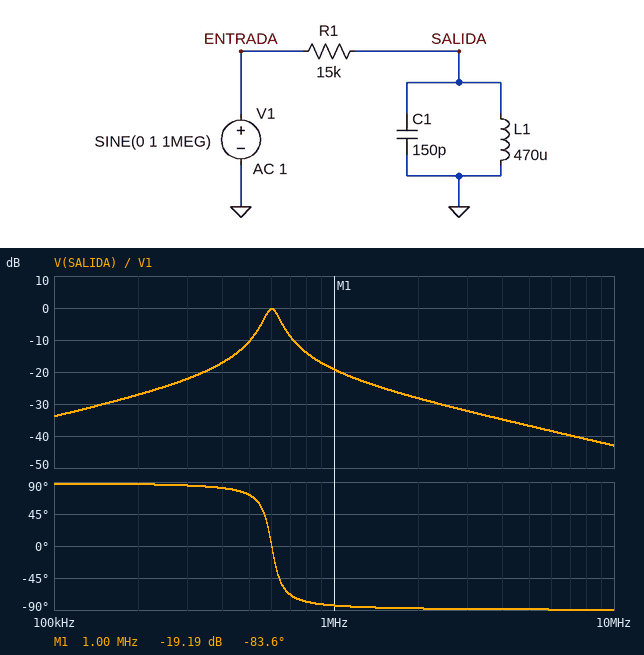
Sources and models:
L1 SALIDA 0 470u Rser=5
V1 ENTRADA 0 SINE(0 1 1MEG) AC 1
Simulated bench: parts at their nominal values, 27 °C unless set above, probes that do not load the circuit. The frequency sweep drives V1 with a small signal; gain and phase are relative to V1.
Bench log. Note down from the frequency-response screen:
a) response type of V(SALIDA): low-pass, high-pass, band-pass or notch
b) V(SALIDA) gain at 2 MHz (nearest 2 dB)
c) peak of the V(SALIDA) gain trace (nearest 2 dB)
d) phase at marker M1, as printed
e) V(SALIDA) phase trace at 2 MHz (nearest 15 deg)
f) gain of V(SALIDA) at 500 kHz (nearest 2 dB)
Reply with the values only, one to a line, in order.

band-pass
-28 dB
0 dB
-83.6 deg
-90 deg
-10 dB
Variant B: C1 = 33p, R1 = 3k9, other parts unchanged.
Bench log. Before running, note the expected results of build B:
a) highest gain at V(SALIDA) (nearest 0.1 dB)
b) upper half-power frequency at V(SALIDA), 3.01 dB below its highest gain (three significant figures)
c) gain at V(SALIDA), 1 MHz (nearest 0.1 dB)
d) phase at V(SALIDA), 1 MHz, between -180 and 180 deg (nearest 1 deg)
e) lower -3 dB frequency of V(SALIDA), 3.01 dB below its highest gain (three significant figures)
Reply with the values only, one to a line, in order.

0 dB
2.04 MHz
-1.0 dB
27 deg
802 kHz
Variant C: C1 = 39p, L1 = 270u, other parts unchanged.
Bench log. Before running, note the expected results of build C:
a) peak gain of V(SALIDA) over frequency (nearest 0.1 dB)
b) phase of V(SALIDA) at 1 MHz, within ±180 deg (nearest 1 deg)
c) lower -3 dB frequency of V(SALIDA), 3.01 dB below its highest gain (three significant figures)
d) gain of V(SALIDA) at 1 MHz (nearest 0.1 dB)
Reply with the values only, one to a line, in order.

-0.1 dB
79 deg
1.42 MHz
-14.4 dB
